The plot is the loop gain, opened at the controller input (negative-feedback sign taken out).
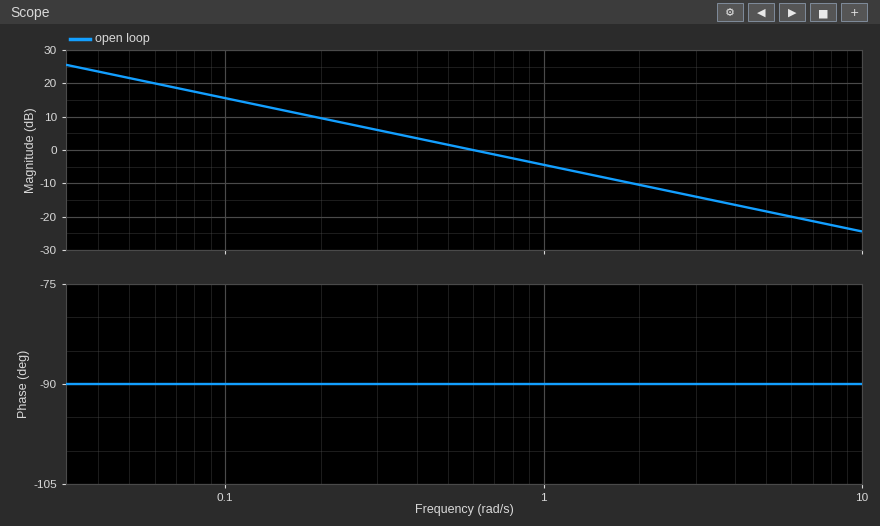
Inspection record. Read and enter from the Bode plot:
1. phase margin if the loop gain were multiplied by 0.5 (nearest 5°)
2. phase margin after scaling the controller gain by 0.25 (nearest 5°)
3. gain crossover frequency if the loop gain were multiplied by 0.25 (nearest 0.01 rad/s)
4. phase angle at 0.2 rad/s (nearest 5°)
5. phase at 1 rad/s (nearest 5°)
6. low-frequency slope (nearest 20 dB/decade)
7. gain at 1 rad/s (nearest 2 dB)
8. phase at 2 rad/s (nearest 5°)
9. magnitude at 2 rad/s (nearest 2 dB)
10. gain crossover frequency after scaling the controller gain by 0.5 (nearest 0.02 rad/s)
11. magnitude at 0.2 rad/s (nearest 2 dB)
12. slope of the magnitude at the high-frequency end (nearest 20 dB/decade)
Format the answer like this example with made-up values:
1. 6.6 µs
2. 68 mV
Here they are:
1. 90°
2. 90°
3. 0.15 rad/s
4. -90°
5. -90°
6. -20 dB/decade
7. -4 dB
8. -90°
9. -10 dB
10. 0.30 rad/s
11. 10 dB
12. -20 dB/decade
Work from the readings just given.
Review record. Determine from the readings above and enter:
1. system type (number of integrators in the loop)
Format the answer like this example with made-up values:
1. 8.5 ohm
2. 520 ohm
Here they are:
1. 1
